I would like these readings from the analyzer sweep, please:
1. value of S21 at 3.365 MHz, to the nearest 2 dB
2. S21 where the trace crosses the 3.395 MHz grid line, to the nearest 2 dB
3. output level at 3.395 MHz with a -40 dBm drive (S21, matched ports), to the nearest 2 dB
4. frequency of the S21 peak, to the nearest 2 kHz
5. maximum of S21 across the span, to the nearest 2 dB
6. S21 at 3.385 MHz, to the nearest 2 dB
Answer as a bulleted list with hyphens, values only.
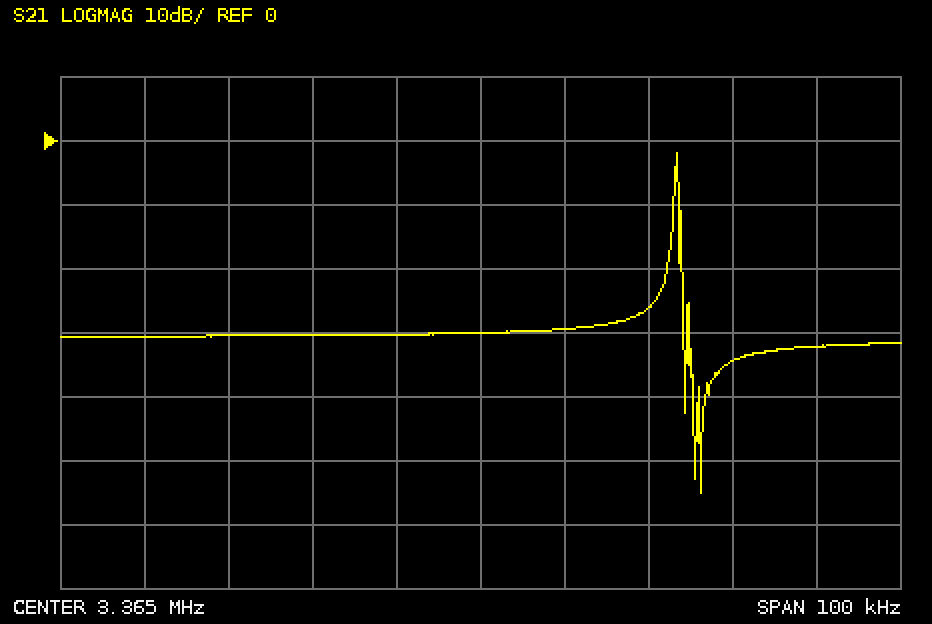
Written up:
- -30 dB
- -34 dB
- -74 dBm
- 3.388 MHz
- -2 dB
- -26 dB
